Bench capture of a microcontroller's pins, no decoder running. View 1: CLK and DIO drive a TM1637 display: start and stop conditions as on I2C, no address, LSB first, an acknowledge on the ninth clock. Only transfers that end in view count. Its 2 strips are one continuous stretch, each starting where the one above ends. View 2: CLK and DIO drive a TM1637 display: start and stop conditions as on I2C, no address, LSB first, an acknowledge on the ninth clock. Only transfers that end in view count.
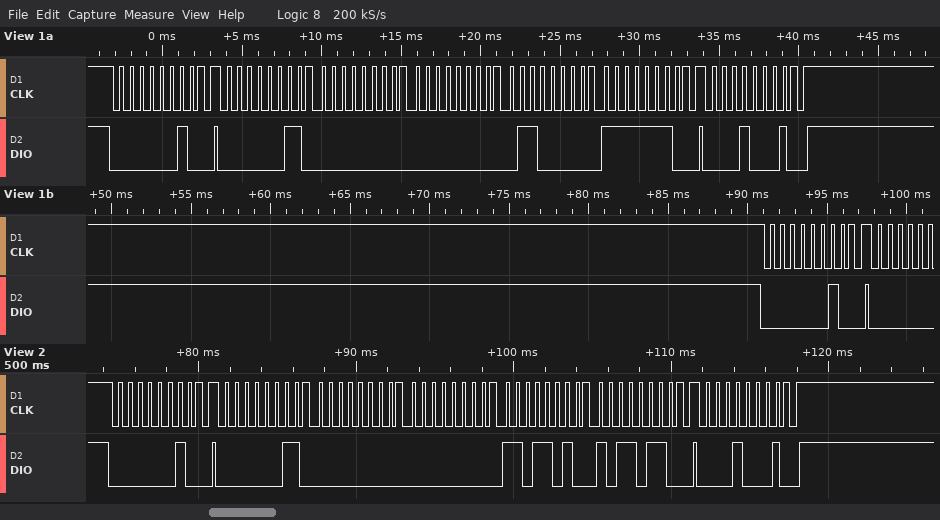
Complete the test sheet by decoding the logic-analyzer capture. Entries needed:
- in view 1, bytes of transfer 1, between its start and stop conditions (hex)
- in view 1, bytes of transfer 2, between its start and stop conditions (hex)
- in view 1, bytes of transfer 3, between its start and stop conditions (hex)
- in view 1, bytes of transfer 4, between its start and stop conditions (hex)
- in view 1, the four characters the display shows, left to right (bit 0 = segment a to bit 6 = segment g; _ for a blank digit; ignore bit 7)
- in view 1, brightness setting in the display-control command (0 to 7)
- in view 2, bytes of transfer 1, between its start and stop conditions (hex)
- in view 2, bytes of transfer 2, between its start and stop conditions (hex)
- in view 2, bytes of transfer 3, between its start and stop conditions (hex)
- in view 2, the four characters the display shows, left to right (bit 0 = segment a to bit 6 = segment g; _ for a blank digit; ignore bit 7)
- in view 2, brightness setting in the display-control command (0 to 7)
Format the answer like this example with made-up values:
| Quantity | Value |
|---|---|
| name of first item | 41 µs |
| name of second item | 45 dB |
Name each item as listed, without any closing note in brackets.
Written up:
| Quantity | Value |
|---|---|
| in view 1, bytes of transfer 1, between its start and stop conditions | 40 |
| in view 1, bytes of transfer 2, between its start and stop conditions | C0 00 00 06 7F |
| in view 1, bytes of transfer 3, between its start and stop conditions | 88 |
| in view 1, bytes of transfer 4, between its start and stop conditions | 40 |
| in view 1, the four characters the display shows, left to right | __18 |
| in view 1, brightness setting in the display-control command | 0 |
| in view 2, bytes of transfer 1, between its start and stop conditions | 40 |
| in view 2, bytes of transfer 2, between its start and stop conditions | C0 00 00 5B 6D |
| in view 2, bytes of transfer 3, between its start and stop conditions | 88 |
| in view 2, the four characters the display shows, left to right | __25 |
| in view 2, brightness setting in the display-control command | 0 |
